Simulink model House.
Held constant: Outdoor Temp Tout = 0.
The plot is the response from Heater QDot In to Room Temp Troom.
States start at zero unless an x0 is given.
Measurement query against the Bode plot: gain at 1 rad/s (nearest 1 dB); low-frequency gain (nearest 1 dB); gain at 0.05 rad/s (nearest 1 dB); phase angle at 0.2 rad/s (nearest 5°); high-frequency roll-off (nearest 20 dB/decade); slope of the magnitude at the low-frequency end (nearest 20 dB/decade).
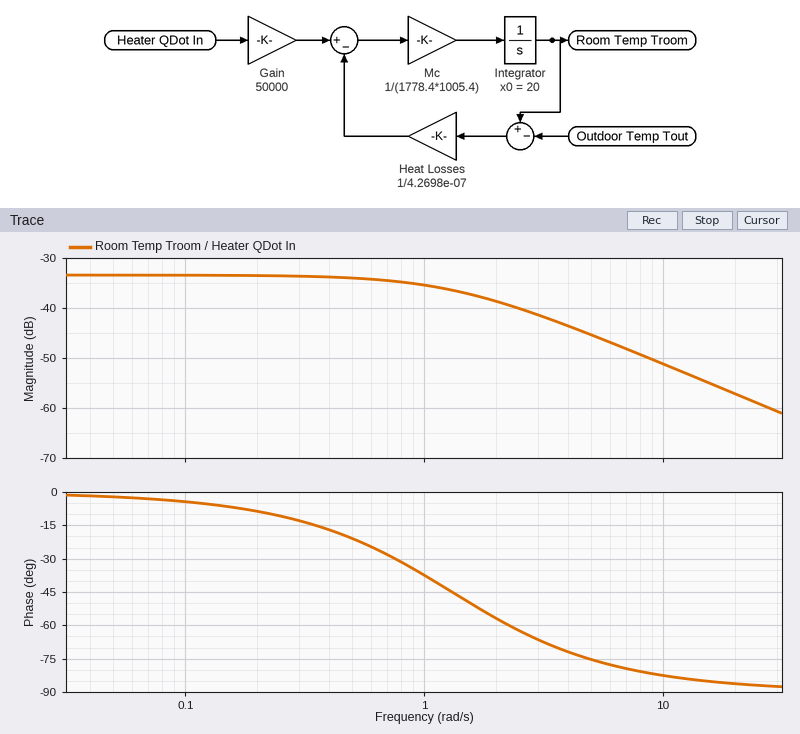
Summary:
-35 dB
-33 dB
-33 dB
-10°
-20 dB/decade
0 dB/decade
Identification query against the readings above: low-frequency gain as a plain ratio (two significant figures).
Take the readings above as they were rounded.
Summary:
0.022
